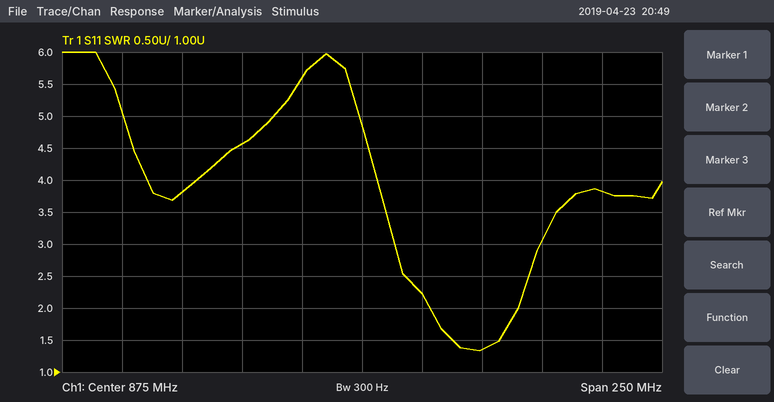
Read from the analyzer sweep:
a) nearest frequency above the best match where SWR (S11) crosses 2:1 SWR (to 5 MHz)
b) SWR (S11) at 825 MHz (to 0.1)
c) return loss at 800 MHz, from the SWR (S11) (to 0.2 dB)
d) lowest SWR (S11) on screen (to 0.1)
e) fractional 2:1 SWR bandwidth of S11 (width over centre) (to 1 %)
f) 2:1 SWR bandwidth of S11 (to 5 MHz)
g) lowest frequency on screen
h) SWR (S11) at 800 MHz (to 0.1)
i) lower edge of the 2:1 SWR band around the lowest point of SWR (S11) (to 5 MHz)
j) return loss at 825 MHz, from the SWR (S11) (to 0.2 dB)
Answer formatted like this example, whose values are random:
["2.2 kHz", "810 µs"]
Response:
["940 MHz", "4.6", "4.6 dB", "1.3", "4 %", "35 MHz", "750 MHz", "3.8", "905 MHz", "3.8 dB"]
